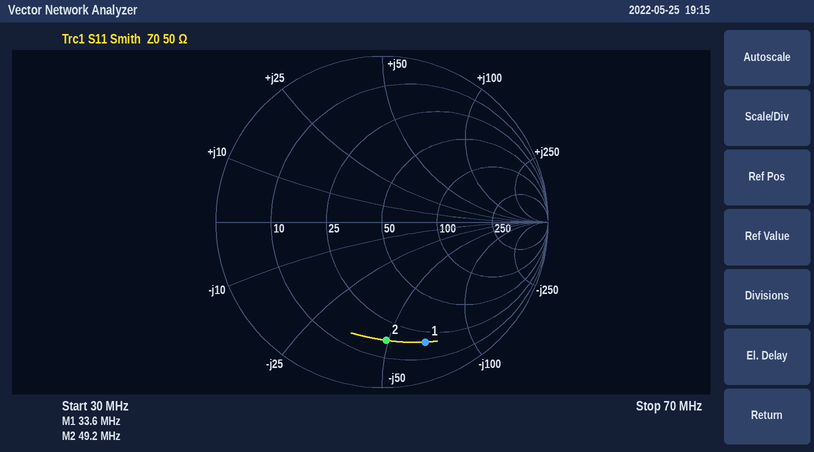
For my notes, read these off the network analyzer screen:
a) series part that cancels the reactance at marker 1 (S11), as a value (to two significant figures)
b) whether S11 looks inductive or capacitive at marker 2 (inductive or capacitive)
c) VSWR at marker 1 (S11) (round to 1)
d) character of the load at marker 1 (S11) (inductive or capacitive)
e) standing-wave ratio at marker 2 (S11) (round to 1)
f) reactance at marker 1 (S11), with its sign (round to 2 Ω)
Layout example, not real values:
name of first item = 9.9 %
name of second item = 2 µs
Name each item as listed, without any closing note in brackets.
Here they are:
series part that cancels the reactance at marker 1 (S11), as a value = 320 nH
whether S11 looks inductive or capacitive at marker 2 = capacitive
VSWR at marker 1 (S11) = 8
character of the load at marker 1 (S11) = capacitive
standing-wave ratio at marker 2 (S11) = 6
reactance at marker 1 (S11), with its sign = -68 Ω
